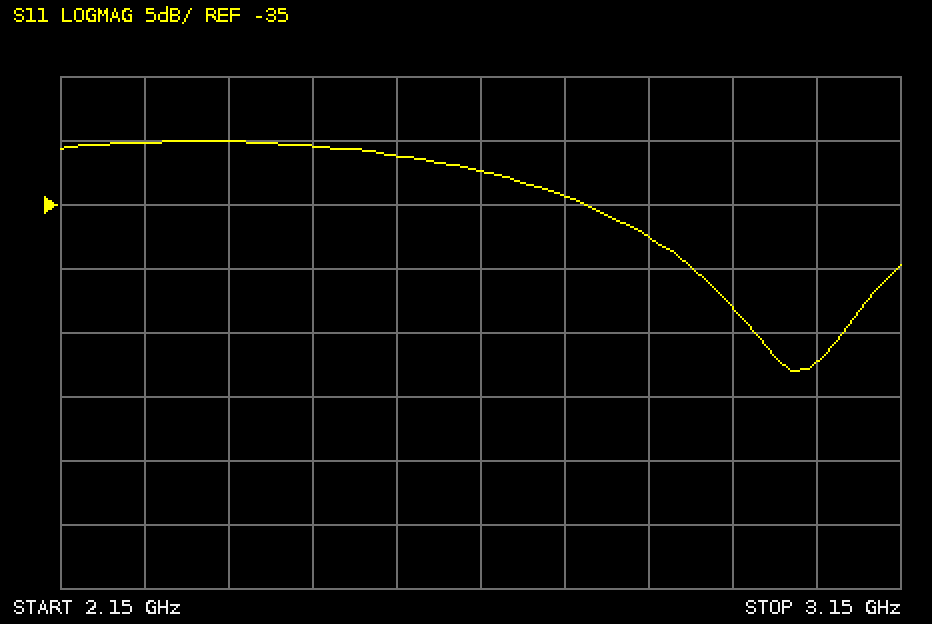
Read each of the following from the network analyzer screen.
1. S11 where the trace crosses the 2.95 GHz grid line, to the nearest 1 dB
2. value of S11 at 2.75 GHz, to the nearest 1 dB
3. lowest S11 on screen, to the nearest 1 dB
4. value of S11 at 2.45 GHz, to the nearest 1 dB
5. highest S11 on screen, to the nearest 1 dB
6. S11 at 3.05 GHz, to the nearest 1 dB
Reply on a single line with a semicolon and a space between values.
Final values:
-43 dB; -34 dB; -48 dB; -30 dB; -30 dB; -47 dB
